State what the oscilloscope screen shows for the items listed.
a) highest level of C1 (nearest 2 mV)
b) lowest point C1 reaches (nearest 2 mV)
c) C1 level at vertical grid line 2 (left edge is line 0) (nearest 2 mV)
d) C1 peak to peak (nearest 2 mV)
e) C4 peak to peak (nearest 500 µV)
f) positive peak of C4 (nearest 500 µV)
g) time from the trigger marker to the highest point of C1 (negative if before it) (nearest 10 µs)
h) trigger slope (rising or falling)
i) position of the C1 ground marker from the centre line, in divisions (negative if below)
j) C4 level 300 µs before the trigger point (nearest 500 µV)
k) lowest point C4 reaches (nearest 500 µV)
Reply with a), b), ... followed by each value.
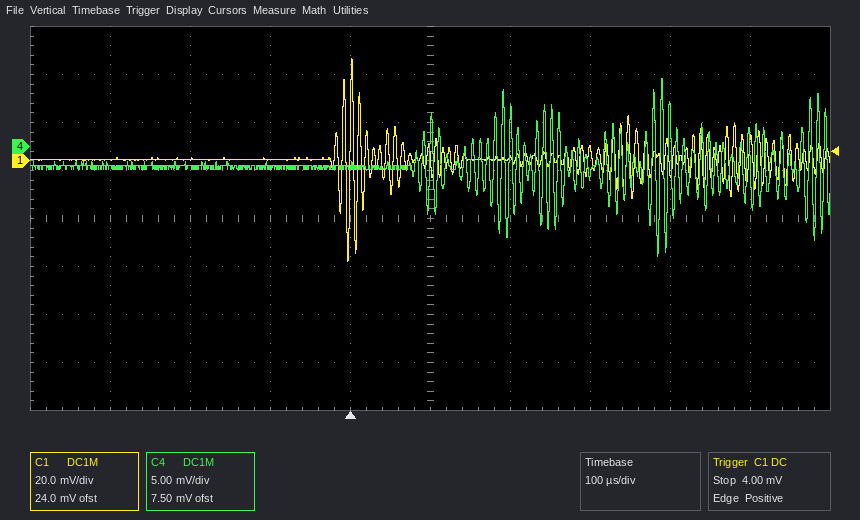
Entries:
a) 42 mV
b) -42 mV
c) 0 mV
d) 84 mV
e) 18.5 mV
f) 7.0 mV
g) 0 µs
h) rising
i) +1.2 div
j) -2.0 mV
k) -11.5 mV
